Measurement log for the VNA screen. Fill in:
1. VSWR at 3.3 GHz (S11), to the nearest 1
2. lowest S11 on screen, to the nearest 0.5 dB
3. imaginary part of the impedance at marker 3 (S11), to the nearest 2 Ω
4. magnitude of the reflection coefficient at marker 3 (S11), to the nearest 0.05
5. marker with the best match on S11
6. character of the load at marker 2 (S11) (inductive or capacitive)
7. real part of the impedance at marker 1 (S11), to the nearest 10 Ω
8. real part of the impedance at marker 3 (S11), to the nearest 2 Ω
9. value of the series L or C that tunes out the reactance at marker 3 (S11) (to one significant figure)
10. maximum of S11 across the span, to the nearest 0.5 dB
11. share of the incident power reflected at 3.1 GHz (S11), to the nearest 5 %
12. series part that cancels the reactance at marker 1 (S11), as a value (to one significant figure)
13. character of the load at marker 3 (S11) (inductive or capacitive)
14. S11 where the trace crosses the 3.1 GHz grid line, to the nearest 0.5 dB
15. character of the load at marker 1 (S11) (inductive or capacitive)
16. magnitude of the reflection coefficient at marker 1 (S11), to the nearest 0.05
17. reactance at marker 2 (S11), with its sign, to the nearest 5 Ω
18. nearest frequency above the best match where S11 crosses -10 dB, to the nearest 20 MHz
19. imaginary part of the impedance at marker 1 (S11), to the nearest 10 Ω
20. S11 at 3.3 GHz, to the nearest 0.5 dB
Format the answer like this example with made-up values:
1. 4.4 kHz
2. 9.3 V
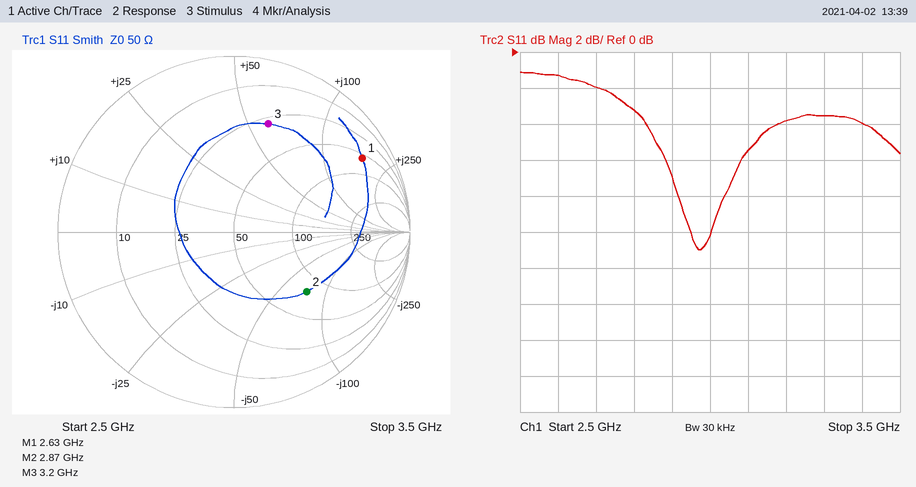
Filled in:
1. 5
2. -11.0 dB
3. +60 Ω
4. 0.65
5. marker 2
6. capacitive
7. 60 Ω
8. 28 Ω
9. 800 fF
10. -1.0 dB
11. 30 %
12. 400 fF
13. inductive
14. -5.5 dB
15. inductive
16. 0.85
17. -75 Ω
18. 3.00 GHz
19. +170 Ω
20. -3.5 dB
